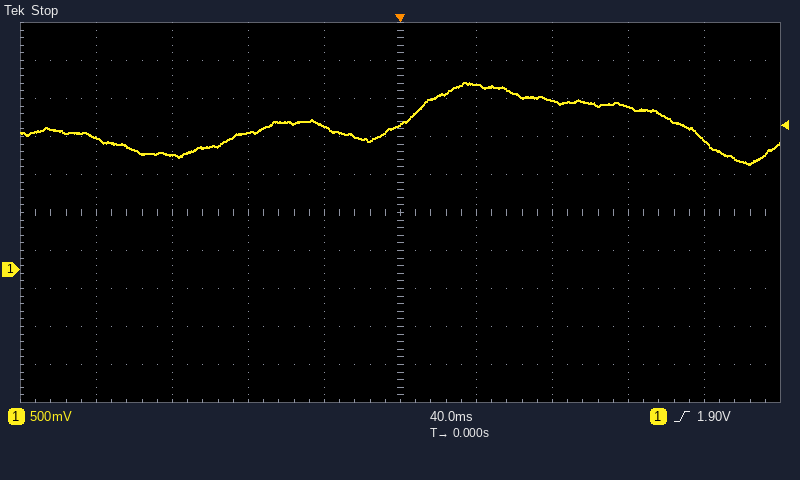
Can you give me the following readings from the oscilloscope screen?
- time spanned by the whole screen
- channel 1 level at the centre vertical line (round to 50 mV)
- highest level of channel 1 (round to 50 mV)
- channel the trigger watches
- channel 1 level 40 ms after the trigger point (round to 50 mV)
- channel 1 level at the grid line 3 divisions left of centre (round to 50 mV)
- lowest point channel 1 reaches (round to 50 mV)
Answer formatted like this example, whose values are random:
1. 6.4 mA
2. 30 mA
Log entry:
1. 400 ms
2. 1.90 V
3. 2.45 V
4. channel 1
5. 2.45 V
6. 1.50 V
7. 1.40 V
